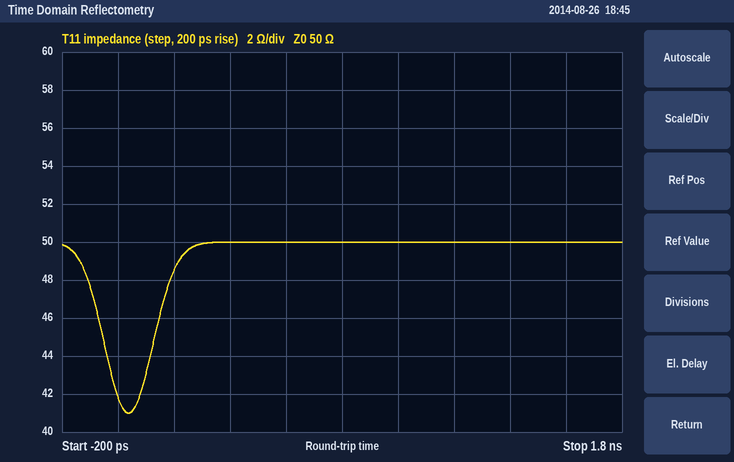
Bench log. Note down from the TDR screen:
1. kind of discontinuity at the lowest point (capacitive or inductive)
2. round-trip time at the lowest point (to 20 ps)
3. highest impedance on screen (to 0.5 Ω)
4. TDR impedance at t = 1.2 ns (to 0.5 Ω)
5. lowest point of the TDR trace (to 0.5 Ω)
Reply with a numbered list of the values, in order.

1. capacitive
2. 40 ps
3. 50.0 Ω
4. 50.0 Ω
5. 41.0 Ω
